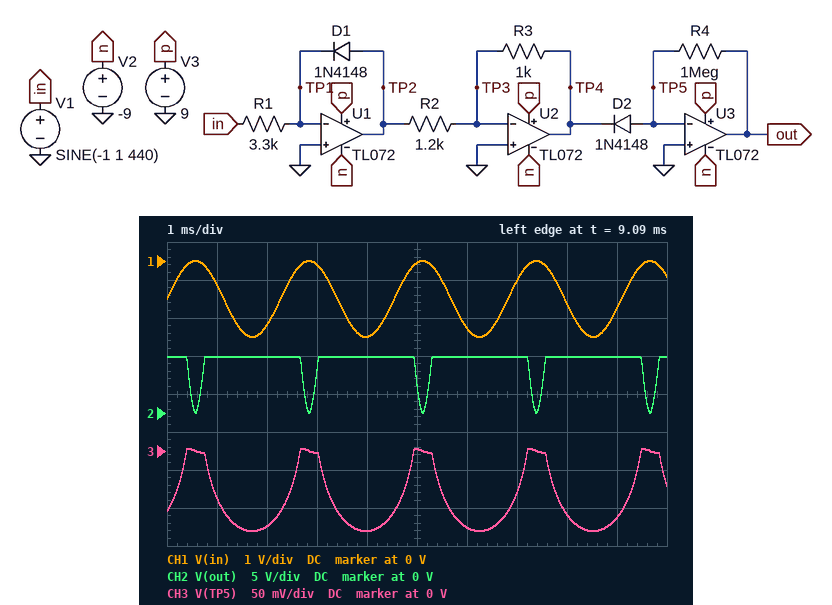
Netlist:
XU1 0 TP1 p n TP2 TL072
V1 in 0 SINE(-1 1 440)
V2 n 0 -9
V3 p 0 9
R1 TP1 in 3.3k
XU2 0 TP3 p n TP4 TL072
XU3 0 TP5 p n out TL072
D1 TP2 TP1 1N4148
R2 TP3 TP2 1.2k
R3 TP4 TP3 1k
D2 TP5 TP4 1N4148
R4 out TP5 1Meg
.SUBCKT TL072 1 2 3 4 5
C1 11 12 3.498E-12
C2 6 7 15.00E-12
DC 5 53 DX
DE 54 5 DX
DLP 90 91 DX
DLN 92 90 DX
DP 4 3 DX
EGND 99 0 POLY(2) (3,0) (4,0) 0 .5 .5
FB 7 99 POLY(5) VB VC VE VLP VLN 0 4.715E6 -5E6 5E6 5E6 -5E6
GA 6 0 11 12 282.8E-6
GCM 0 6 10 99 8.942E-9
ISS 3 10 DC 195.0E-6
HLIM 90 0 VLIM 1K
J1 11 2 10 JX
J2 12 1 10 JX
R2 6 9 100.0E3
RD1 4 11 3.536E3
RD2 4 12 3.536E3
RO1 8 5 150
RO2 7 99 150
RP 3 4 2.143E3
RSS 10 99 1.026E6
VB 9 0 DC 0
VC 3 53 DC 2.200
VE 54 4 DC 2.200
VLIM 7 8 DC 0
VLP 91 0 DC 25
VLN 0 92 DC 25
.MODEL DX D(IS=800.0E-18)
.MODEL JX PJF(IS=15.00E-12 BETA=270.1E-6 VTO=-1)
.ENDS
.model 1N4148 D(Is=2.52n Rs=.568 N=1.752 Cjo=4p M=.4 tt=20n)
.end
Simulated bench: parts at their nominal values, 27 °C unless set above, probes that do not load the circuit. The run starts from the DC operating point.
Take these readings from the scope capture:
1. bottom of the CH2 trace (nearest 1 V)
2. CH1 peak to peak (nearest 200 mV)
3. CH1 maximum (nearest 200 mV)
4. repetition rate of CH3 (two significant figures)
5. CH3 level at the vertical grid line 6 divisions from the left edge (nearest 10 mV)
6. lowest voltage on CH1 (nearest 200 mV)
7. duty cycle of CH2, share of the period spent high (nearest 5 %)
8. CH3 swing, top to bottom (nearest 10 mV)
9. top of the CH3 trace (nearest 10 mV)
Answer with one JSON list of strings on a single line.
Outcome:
["0 V", "2.0 V", "0 V", "440 Hz", "-100 mV", "-2.0 V", "90 %", "110 mV", "0 V"]
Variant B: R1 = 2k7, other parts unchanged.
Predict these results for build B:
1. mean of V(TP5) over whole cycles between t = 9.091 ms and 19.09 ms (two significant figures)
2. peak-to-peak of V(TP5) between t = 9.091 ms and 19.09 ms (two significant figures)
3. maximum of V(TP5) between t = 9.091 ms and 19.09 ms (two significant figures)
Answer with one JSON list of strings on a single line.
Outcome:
["-72 mV", "120 mV", "3.3 mV"]
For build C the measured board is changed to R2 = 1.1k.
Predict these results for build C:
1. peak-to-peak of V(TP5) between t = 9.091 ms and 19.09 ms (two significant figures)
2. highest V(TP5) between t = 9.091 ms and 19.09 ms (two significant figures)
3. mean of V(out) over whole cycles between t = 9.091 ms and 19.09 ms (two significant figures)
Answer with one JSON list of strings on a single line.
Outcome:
["150 mV", "4.8 mV", "6.9 V"]
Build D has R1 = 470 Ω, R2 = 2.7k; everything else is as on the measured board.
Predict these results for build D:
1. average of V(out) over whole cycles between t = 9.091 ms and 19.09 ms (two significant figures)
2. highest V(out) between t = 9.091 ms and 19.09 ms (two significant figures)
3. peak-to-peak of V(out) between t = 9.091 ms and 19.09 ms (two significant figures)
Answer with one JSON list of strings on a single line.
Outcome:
["360 mV", "520 mV", "510 mV"]
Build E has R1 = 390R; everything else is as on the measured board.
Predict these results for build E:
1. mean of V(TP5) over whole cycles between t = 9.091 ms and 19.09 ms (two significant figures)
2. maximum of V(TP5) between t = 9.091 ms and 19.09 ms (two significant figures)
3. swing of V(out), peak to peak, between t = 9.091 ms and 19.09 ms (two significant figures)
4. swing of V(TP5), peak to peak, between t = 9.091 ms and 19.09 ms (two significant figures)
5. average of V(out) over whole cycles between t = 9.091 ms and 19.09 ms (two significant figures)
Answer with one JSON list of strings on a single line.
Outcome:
["-140 mV", "8.7 mV", "7.3 V", "200 mV", "7.2 V"]
